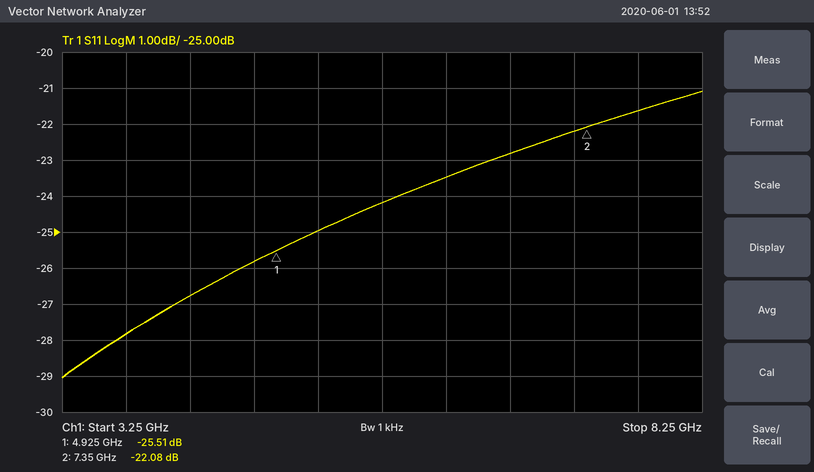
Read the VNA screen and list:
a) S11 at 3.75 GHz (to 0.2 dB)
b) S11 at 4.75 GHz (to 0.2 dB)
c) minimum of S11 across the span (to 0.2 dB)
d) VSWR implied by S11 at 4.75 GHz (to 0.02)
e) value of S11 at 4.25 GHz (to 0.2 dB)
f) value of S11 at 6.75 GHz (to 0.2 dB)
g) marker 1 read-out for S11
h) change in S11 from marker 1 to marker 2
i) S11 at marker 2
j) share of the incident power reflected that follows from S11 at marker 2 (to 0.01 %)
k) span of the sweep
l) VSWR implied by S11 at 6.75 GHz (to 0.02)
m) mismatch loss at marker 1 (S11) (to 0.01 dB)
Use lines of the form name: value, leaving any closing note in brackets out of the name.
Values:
S11 at 3.75 GHz: -27.8 dB
S11 at 4.75 GHz: -25.8 dB
minimum of S11 across the span: -29.0 dB
VSWR implied by S11 at 4.75 GHz: 1.10
value of S11 at 4.25 GHz: -26.8 dB
value of S11 at 6.75 GHz: -22.8 dB
marker 1 read-out for S11: -25.51 dB
change in S11 from marker 1 to marker 2: 3.43 dB
S11 at marker 2: -22.08 dB
share of the incident power reflected that follows from S11 at marker 2: 0.62 %
span of the sweep: 5 GHz
VSWR implied by S11 at 6.75 GHz: 1.16
mismatch loss at marker 1 (S11): 0.01 dB
